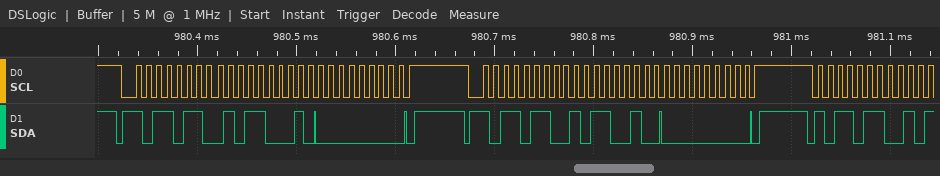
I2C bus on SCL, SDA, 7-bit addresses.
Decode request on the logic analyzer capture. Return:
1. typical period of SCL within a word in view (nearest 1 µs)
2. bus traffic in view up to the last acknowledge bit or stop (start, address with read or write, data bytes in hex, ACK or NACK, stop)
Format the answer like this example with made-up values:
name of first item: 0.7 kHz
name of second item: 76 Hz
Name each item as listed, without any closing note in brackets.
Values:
typical period of SCL within a word in view: 10 µs
bus traffic in view up to the last acknowledge bit or stop: start, address 5B write ACK, B1 ACK, 00 ACK, stop, start, address 5B write ACK, B2 ACK, 00 ACK, stop, start, address 5B write ACK
